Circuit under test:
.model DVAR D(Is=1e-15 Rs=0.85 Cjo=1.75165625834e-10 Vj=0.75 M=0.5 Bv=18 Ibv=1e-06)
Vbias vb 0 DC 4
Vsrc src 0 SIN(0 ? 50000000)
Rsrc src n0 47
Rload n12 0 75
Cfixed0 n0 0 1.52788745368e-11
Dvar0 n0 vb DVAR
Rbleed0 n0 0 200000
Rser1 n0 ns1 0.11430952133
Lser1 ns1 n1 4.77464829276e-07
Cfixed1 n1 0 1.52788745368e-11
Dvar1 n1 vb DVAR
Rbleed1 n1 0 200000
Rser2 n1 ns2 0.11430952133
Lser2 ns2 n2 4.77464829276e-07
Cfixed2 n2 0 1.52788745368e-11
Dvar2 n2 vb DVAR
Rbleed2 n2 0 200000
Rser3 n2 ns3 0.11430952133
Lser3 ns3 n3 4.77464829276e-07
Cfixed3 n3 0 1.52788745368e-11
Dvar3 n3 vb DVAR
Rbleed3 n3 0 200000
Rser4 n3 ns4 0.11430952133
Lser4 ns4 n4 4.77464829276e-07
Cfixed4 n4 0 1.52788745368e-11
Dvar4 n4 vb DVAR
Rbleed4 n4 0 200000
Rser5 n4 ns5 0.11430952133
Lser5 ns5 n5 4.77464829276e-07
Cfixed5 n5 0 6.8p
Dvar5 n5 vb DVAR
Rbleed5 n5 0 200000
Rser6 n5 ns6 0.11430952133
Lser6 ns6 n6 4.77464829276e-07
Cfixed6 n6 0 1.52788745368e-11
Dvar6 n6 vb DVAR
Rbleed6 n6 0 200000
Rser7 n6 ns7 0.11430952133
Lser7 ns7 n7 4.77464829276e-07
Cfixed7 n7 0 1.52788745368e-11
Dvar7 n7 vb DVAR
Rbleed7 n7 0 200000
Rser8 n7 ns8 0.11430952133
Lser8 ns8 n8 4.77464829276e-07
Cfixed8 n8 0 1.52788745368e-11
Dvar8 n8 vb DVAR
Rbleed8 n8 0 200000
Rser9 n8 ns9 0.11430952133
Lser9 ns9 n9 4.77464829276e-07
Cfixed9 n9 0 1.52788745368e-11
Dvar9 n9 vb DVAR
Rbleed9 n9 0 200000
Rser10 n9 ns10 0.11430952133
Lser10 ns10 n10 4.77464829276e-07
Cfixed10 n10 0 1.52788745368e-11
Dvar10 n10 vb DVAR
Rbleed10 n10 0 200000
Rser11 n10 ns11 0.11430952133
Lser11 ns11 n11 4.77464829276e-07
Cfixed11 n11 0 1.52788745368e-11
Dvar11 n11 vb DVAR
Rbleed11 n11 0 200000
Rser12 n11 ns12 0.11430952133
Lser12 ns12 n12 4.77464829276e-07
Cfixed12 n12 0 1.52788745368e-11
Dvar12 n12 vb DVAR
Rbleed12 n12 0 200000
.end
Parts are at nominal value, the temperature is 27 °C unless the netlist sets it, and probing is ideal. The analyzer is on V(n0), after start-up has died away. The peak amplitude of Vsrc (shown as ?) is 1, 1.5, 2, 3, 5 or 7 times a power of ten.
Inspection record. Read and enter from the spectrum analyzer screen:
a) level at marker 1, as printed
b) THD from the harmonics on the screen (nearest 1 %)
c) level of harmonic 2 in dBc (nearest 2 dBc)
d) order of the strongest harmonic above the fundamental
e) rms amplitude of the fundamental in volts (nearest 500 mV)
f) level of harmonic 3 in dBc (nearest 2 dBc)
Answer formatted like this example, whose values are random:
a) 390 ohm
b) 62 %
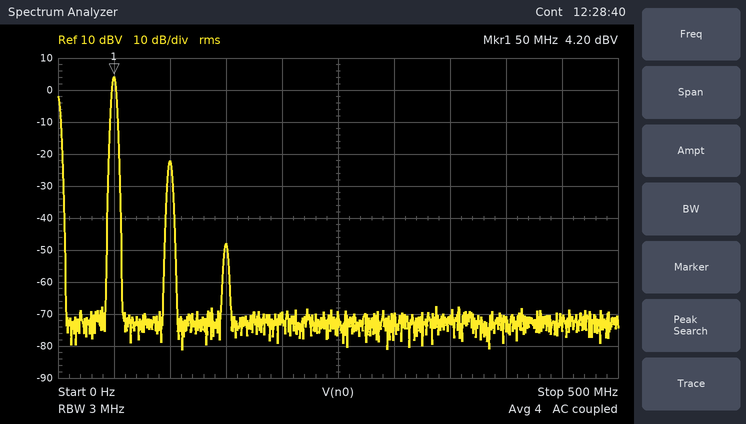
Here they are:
a) 4.20 dBV
b) 5 %
c) -26 dBc
d) 2
e) 1.5 V
f) -52 dBc
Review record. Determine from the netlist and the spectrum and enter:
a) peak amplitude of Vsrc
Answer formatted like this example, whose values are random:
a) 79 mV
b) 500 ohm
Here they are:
a) 3 V
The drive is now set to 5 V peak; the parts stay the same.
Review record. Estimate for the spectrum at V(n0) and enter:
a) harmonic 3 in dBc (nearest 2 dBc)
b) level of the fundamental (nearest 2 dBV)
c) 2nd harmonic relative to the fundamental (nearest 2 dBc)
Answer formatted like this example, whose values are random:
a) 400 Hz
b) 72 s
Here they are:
a) -42 dBc
b) 8 dBV
c) -22 dBc
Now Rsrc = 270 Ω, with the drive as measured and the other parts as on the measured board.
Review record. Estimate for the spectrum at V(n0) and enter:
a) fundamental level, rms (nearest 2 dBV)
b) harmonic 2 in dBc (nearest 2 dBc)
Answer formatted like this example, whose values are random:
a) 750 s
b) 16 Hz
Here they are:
a) -6 dBV
b) -36 dBc
